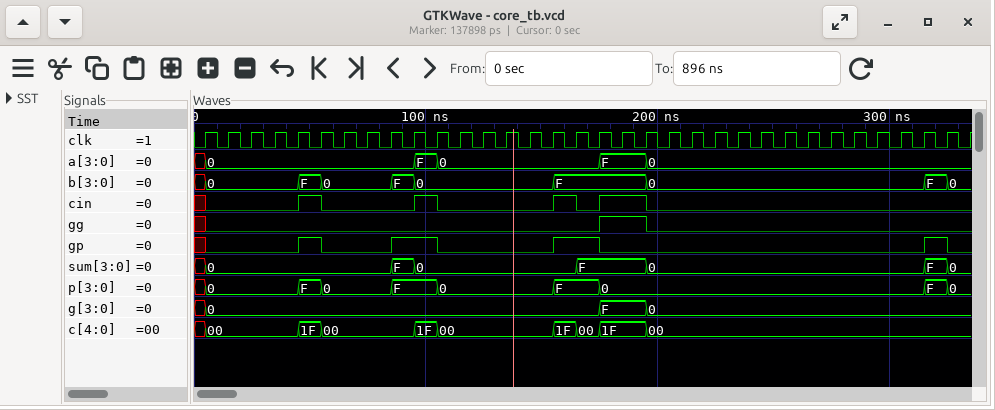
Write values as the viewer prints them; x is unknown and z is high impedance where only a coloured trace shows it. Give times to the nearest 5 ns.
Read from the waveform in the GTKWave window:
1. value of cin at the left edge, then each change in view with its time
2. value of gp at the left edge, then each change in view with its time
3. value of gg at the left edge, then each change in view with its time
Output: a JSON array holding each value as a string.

["x, 0 at 5 ns, 1 at 45 ns, 0 at 55 ns, 1 at 95 ns, 0 at 105 ns, 1 at 155 ns, 0 at 165 ns, 1 at 175 ns, 0 at 195 ns", "x, 0 at 5 ns, 1 at 45 ns, 0 at 55 ns, 1 at 85 ns, 0 at 105 ns, 1 at 155 ns, 0 at 175 ns, 1 at 315 ns, 0 at 325 ns", "x, 0 at 5 ns, 1 at 175 ns, 0 at 195 ns"]
